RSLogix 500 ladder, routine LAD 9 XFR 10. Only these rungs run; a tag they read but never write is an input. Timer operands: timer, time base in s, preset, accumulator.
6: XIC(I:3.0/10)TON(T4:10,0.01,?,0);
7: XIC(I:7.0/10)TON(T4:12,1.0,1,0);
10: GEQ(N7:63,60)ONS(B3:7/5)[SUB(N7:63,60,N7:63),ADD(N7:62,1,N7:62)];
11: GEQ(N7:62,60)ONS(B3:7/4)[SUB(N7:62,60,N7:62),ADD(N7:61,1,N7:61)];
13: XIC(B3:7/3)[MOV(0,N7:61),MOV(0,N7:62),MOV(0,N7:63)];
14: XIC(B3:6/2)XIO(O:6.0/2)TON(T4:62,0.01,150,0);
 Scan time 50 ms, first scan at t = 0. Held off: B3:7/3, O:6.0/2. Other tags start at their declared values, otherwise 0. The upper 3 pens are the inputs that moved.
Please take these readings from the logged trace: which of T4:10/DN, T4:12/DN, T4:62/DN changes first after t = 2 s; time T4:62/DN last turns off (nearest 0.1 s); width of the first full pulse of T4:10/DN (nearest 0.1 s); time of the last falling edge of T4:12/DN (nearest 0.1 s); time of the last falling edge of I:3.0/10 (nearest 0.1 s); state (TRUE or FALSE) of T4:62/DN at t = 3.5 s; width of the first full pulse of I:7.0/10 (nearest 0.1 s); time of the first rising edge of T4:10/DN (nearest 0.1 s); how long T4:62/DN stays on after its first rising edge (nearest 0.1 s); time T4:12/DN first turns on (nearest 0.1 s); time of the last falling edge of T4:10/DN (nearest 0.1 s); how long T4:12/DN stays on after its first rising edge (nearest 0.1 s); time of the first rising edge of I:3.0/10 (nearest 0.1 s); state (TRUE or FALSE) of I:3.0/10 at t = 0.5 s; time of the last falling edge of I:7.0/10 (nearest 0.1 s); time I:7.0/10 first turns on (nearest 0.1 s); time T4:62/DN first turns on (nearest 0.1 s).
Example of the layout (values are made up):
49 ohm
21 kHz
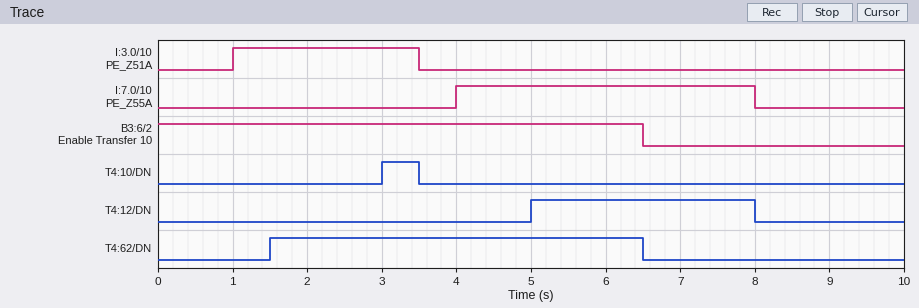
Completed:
T4:10/DN
6.5 s
0.5 s
8.0 s
3.5 s
TRUE
4.0 s
3.0 s
5.0 s
5.0 s
3.5 s
3.0 s
1.0 s
FALSE
8.0 s
4.0 s
1.5 s
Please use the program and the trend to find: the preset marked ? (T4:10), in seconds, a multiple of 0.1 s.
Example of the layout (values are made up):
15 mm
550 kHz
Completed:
2.0 s
